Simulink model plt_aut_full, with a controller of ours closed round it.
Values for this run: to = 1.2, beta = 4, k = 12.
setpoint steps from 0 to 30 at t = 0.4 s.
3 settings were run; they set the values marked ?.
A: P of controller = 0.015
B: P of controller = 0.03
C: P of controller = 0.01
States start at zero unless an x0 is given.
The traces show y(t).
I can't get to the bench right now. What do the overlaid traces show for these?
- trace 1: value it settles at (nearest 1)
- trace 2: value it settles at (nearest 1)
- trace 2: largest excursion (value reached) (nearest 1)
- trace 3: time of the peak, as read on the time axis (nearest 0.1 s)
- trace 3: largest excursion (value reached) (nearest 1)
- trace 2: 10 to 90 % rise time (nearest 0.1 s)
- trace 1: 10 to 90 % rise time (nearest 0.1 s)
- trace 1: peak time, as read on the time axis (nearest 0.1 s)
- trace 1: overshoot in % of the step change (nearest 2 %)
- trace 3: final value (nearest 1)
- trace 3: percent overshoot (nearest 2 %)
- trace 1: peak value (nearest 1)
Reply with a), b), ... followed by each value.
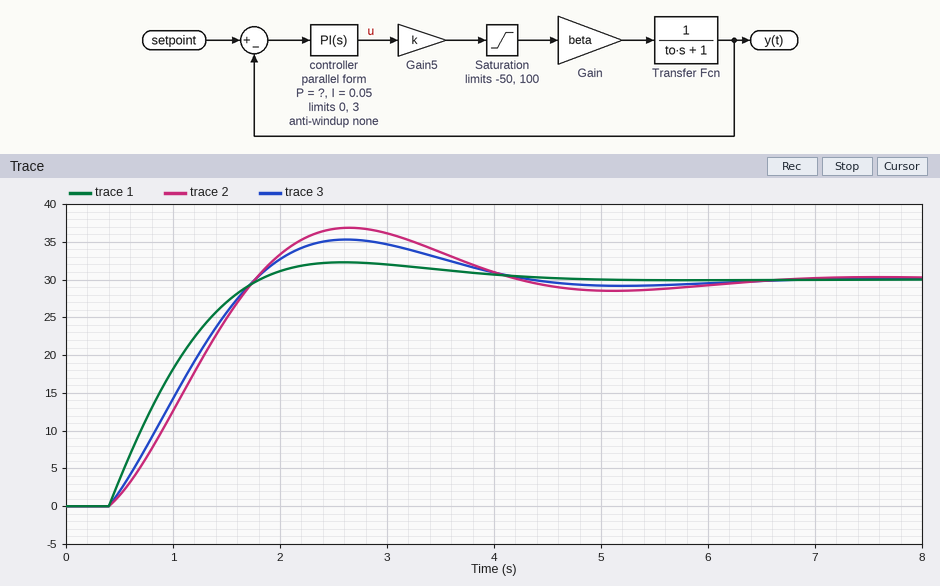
a) 30
b) 30
c) 37
d) 2.6 s
e) 35
f) 1.0 s
g) 1.0 s
h) 2.6 s
i) 8 %
j) 30
k) 18 %
l) 32
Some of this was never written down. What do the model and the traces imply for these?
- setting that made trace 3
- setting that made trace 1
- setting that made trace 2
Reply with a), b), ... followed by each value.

a) A
b) B
c) C
